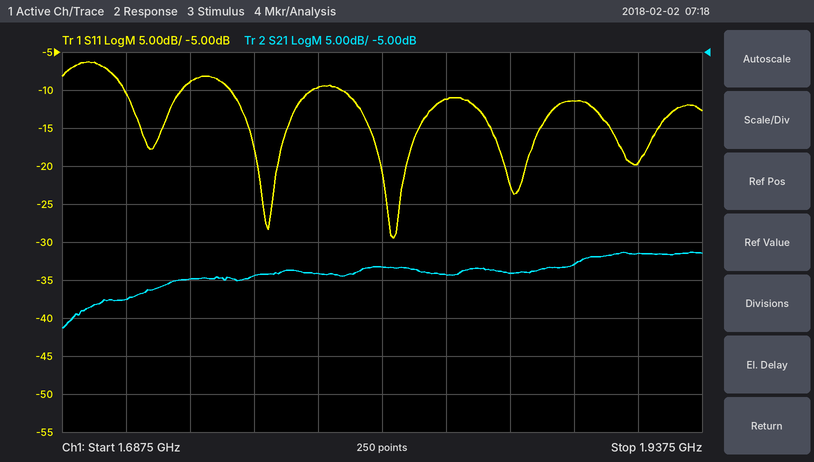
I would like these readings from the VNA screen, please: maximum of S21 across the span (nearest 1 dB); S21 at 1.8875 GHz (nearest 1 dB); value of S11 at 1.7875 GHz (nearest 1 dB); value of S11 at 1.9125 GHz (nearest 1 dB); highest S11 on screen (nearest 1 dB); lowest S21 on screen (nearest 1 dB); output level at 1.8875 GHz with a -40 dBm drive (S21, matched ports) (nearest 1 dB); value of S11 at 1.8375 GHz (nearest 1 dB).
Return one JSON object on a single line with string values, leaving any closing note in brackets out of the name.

{"maximum of S21 across the span": "-31 dB", "S21 at 1.8875 GHz": "-33 dB", "value of S11 at 1.7875 GHz": "-10 dB", "value of S11 at 1.9125 GHz": "-20 dB", "highest S11 on screen": "-6 dB", "lowest S21 on screen": "-41 dB", "output level at 1.8875 GHz with a -40 dBm drive (S21, matched ports)": "-73 dBm", "value of S11 at 1.8375 GHz": "-11 dB"}
